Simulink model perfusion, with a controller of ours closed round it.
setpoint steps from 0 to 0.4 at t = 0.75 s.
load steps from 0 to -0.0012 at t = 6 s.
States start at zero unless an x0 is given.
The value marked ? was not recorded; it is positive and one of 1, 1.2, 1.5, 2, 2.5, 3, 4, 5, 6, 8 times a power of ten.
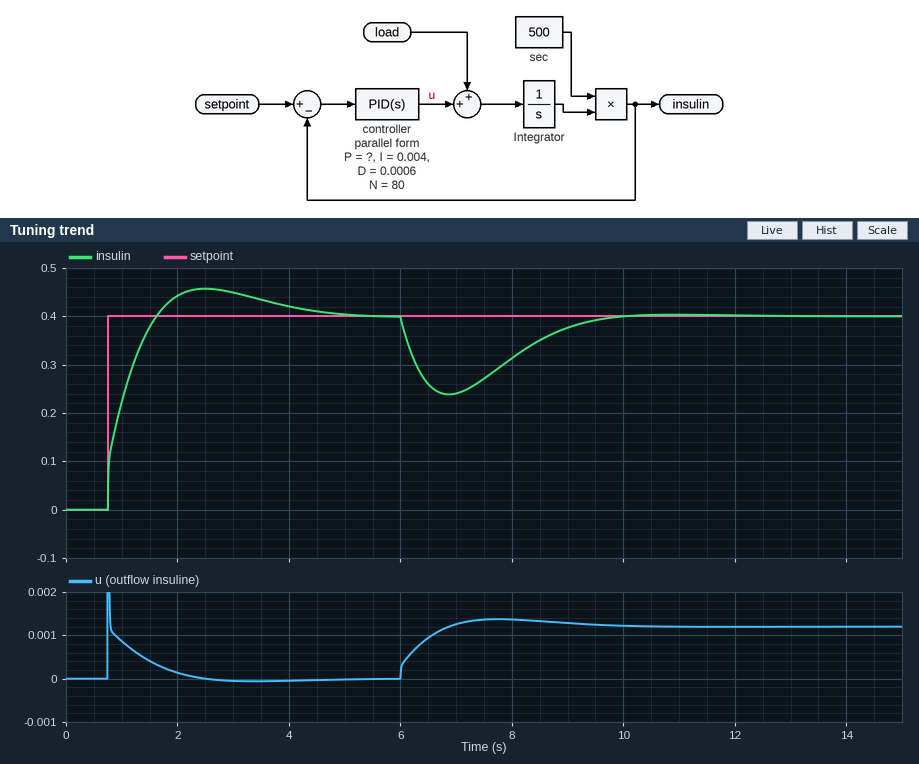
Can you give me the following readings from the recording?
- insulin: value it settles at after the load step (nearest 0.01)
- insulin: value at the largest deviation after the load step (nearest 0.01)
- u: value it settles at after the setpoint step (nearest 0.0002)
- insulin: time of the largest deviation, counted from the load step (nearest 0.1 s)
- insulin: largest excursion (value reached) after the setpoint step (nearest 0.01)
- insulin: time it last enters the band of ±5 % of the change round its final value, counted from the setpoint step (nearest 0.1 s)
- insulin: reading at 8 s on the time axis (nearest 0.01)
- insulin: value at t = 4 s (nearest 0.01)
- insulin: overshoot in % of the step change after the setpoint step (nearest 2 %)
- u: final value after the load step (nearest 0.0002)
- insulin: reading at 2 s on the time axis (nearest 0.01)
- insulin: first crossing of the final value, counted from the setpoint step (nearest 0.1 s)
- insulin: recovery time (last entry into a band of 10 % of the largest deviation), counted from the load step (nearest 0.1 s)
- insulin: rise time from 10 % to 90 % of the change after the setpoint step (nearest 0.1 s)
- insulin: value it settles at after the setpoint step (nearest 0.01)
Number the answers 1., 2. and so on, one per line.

1. 0.40
2. 0.24
3. 0.0000
4. 0.9 s
5. 0.46
6. 3.3 s
7. 0.31
8. 0.42
9. 14 %
10. 0.0012
11. 0.44
12. 0.9 s
13. 3.2 s
14. 0.7 s
15. 0.40
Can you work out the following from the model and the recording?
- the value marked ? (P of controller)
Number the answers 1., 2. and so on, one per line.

1. 0.005
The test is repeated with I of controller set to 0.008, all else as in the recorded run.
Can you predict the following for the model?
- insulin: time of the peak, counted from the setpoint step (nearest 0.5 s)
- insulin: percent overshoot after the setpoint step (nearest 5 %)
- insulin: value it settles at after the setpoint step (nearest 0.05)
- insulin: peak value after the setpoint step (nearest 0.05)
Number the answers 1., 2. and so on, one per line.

1. 1.5 s
2. 20 %
3. 0.40
4. 0.50
